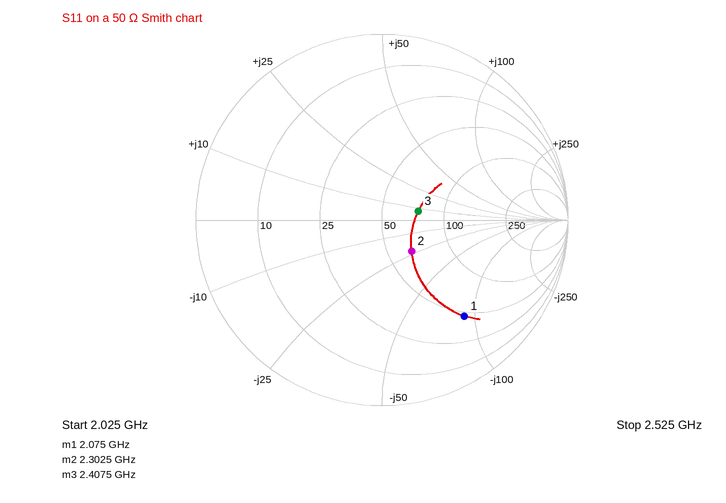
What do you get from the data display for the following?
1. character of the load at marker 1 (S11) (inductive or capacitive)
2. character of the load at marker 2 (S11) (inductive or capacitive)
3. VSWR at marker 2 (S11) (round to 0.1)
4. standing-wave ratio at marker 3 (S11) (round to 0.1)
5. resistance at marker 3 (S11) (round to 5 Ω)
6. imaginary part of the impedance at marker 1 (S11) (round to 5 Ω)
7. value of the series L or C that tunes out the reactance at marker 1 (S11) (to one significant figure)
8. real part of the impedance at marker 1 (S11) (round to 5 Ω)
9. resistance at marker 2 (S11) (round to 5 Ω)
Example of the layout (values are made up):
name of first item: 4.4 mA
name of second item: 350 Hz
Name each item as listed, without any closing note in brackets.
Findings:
character of the load at marker 1 (S11): capacitive
character of the load at marker 2 (S11): capacitive
VSWR at marker 2 (S11): 1.6
standing-wave ratio at marker 3 (S11): 1.5
resistance at marker 3 (S11): 75 Ω
imaginary part of the impedance at marker 1 (S11): -90 Ω
value of the series L or C that tunes out the reactance at marker 1 (S11): 7 nH
real part of the impedance at marker 1 (S11): 45 Ω
resistance at marker 2 (S11): 65 Ω
